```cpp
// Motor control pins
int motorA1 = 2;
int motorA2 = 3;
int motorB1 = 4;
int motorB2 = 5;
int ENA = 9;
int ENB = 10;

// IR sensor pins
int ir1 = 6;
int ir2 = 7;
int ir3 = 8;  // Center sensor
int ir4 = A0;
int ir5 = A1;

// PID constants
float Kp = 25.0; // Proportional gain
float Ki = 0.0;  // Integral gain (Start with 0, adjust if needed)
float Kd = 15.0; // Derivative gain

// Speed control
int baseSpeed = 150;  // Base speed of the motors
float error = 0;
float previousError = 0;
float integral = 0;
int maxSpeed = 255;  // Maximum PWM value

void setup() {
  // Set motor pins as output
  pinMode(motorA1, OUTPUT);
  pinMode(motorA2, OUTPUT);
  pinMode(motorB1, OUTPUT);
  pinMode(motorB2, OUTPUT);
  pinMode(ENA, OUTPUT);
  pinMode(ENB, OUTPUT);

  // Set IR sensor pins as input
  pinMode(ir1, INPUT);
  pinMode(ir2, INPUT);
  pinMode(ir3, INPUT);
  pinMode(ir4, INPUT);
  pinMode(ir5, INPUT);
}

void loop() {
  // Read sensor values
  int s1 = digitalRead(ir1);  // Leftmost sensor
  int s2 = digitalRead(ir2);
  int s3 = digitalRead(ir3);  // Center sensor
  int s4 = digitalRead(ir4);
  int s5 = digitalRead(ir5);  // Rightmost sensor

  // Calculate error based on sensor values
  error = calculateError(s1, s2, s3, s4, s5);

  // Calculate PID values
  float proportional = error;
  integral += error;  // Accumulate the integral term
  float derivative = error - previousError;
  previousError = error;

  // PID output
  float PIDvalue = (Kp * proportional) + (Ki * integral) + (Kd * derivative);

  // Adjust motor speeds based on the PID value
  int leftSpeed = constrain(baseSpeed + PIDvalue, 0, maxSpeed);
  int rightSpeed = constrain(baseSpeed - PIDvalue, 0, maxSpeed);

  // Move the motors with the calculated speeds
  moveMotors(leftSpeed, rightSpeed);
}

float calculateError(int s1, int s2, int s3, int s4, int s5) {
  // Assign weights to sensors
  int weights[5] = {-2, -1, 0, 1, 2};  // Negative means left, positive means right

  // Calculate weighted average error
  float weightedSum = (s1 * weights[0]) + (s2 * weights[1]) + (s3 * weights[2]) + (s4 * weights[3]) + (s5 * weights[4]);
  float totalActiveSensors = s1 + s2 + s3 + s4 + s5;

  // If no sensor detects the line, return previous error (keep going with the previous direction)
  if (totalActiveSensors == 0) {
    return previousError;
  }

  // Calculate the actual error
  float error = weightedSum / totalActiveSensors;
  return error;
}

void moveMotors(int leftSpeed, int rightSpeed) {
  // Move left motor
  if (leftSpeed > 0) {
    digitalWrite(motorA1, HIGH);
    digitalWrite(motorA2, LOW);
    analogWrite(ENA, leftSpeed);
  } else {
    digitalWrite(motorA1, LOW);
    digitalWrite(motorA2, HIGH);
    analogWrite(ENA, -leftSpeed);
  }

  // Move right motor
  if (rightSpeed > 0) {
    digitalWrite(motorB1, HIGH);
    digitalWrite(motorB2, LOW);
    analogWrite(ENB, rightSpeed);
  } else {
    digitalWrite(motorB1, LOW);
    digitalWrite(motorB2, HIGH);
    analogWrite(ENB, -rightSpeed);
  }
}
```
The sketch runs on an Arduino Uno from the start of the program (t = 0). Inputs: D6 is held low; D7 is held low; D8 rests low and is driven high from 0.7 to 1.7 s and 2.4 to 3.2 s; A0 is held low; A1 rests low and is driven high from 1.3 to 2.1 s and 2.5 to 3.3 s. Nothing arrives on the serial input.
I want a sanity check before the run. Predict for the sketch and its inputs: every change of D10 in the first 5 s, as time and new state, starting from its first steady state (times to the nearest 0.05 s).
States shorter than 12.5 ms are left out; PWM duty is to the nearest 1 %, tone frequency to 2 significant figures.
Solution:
0 s PWM 59 %; 1.3 s PWM 49 %; 1.7 s PWM 39 %; 2.4 s PWM 59 %; 2.5 s PWM 49 %; 3.2 s PWM 39 %
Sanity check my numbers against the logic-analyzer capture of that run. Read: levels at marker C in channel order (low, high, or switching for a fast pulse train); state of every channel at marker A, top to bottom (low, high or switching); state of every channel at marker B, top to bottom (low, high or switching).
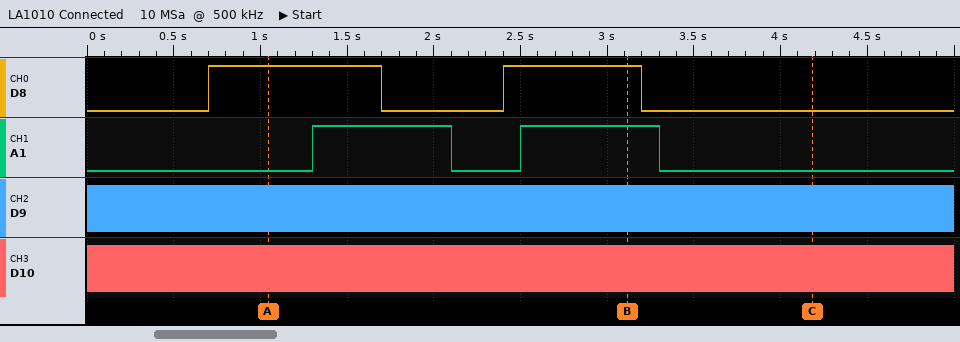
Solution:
D8 low, A1 low, D9 switching, D10 switching
D8 high, A1 low, D9 switching, D10 switching
D8 high, A1 high, D9 switching, D10 switching
